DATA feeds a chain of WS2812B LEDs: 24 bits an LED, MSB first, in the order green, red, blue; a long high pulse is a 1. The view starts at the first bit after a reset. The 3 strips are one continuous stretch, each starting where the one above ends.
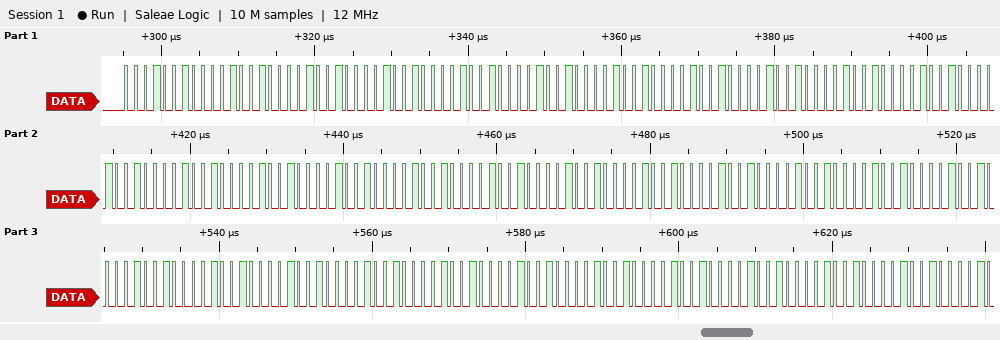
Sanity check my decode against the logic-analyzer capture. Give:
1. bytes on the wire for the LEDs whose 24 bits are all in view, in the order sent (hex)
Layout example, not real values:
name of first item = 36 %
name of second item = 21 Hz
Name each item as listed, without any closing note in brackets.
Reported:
bytes on the wire for the LEDs whose 24 bits are all in view, in the order sent = 12 12 12 12 12 12 12 12 12 12 12 12 12 12 12 12 12 12 12 12 12 12 12 12 12 12 12 12 12 12 12 12 12
